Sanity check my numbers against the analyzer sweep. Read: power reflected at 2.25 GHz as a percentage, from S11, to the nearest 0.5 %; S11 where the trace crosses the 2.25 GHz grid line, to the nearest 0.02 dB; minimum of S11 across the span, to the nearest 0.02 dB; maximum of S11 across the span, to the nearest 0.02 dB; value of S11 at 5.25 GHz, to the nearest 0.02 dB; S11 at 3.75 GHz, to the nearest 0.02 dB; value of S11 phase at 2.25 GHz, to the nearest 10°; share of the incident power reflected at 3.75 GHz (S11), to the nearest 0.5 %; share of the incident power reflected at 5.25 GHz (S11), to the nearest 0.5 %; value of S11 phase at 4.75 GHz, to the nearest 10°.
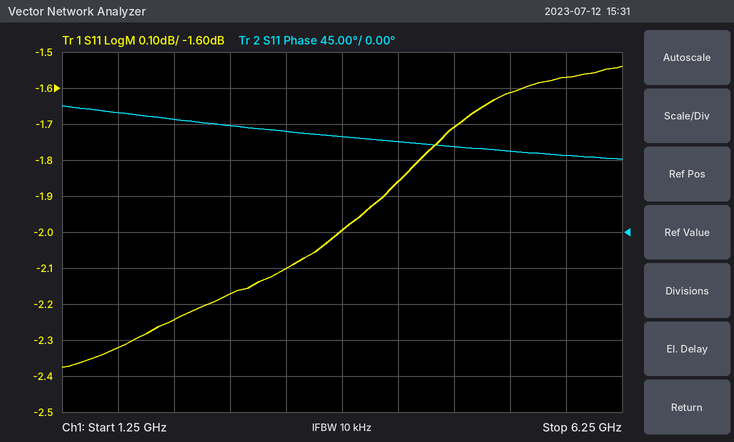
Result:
59.5 %
-2.24 dB
-2.38 dB
-1.54 dB
-1.62 dB
-2.00 dB
140°
63.0 %
69.0 %
110°
